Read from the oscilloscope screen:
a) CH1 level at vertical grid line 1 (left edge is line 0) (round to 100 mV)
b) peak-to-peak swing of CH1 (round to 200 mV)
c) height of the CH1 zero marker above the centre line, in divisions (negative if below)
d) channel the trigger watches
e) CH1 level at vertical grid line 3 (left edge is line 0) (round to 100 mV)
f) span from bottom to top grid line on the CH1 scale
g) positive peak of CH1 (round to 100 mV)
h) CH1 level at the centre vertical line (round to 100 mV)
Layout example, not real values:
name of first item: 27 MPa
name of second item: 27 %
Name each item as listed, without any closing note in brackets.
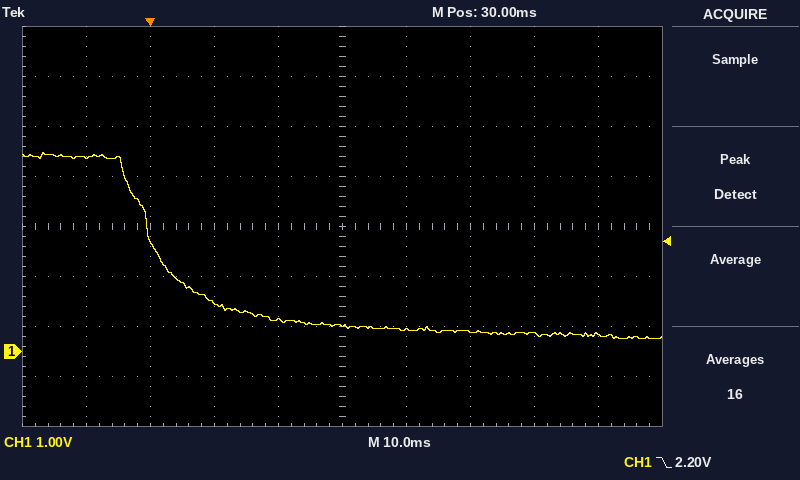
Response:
CH1 level at vertical grid line 1 (left edge is line 0): 3.9 V
peak-to-peak swing of CH1: 3.8 V
height of the CH1 zero marker above the centre line, in divisions: -2.5 div
channel the trigger watches: CH1
CH1 level at vertical grid line 3 (left edge is line 0): 1.0 V
span from bottom to top grid line on the CH1 scale: 8 V
positive peak of CH1: 4.0 V
CH1 level at the centre vertical line: 500 mV
